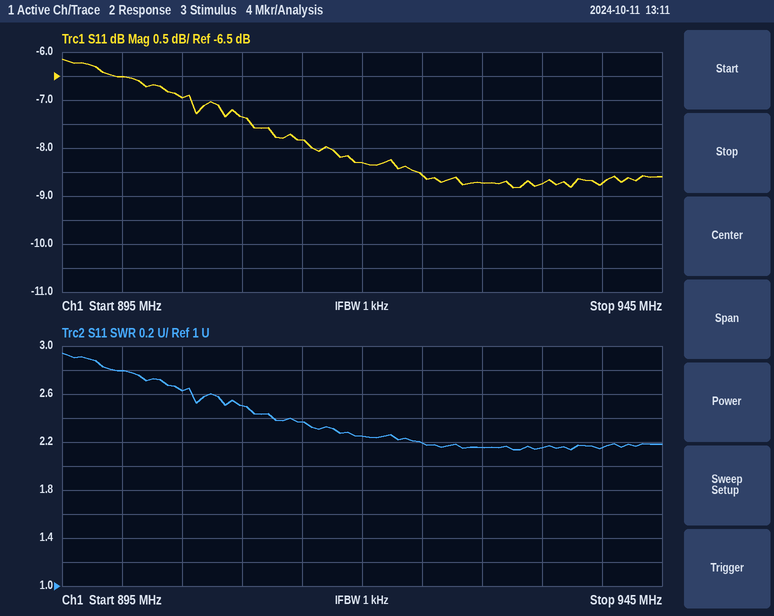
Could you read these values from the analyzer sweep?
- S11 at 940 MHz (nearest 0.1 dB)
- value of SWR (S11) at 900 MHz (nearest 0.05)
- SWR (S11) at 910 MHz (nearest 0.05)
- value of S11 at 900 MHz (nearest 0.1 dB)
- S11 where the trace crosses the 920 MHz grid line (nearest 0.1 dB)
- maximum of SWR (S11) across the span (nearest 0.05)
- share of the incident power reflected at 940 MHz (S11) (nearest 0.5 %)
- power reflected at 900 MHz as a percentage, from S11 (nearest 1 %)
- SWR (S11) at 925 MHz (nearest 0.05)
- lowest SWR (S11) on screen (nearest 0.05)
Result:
-8.7 dB
2.80
2.50
-6.5 dB
-8.3 dB
2.95
13.5 %
22 %
2.20
2.15
